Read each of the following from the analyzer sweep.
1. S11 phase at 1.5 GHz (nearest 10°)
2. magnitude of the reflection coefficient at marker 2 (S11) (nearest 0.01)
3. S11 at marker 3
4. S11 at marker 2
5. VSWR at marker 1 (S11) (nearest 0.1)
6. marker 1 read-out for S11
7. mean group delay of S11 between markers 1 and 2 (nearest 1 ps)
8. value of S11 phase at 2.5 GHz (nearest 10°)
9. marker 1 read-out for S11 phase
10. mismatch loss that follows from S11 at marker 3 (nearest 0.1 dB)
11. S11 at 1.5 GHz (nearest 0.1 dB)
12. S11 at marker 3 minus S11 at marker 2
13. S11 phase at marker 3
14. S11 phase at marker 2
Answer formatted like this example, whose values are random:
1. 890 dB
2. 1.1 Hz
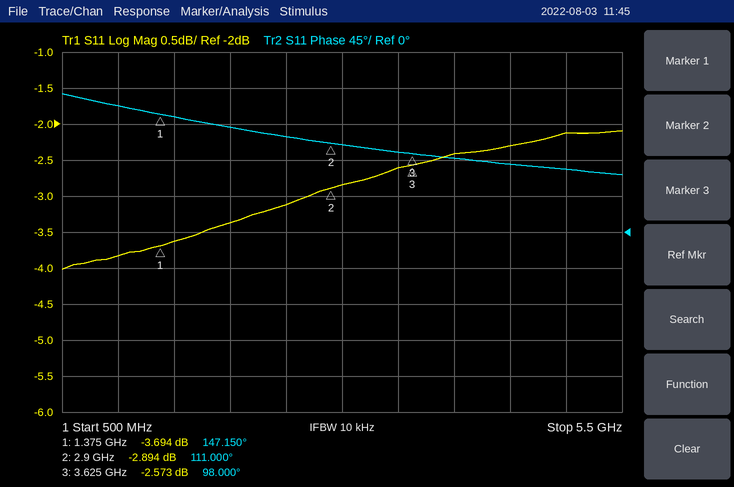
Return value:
1. 140°
2. 0.72
3. -2.573 dB
4. -2.894 dB
5. 4.8
6. -3.694 dB
7. 66 ps
8. 120°
9. 147.150°
10. 3.5 dB
11. -3.6 dB
12. 0.321 dB
13. 98.000°
14. 111.000°
